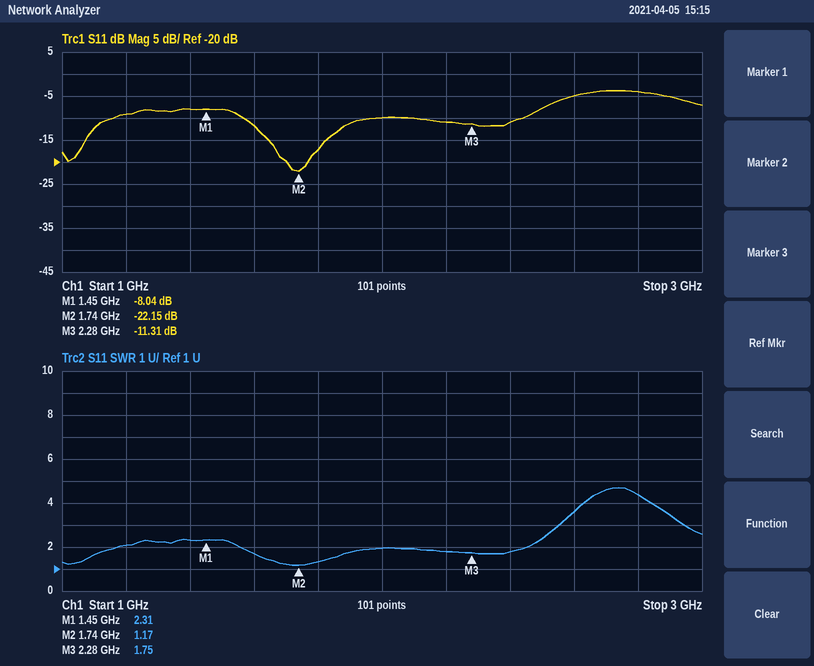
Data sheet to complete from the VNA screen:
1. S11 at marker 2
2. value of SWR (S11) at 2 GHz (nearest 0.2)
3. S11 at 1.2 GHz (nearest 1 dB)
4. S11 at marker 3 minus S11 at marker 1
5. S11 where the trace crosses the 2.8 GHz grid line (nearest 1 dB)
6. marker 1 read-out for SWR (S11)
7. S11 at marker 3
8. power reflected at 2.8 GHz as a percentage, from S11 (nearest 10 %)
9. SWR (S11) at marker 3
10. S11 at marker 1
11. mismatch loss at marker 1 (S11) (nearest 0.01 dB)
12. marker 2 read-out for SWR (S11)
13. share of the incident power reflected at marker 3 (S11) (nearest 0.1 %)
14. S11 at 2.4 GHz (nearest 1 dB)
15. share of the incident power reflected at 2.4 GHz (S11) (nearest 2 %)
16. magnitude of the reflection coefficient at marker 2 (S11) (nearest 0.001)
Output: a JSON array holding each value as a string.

["-22.15 dB", "2.0", "-9 dB", "-3.27 dB", "-4 dB", "2.31", "-11.31 dB", "40 %", "1.75", "-8.04 dB", "0.74 dB", "1.17", "7.4 %", "-11 dB", "8 %", "0.078"]
